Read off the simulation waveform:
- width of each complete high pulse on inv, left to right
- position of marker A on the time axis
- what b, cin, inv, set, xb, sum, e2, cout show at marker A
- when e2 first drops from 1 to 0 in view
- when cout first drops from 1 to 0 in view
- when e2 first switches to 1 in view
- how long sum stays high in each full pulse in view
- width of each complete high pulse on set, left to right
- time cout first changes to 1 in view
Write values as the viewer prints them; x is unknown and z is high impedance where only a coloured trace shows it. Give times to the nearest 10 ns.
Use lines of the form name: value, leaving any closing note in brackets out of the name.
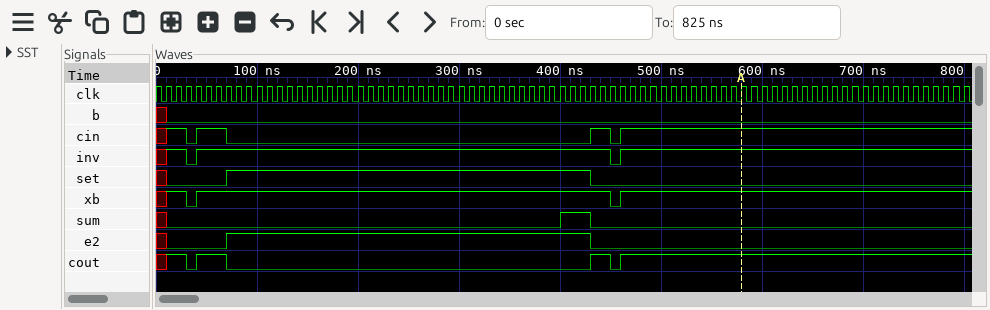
width of each complete high pulse on inv, left to right: 410 ns
position of marker A on the time axis: 580 ns
what b, cin, inv, set, xb, sum, e2, cout show at marker A: b=0, cin=1, inv=1, set=0, xb=1, sum=0, e2=0, cout=1
when e2 first drops from 1 to 0 in view: 430 ns
when cout first drops from 1 to 0 in view: 30 ns
when e2 first switches to 1 in view: 70 ns
how long sum stays high in each full pulse in view: 30 ns
width of each complete high pulse on set, left to right: 360 ns
time cout first changes to 1 in view: 10 ns
